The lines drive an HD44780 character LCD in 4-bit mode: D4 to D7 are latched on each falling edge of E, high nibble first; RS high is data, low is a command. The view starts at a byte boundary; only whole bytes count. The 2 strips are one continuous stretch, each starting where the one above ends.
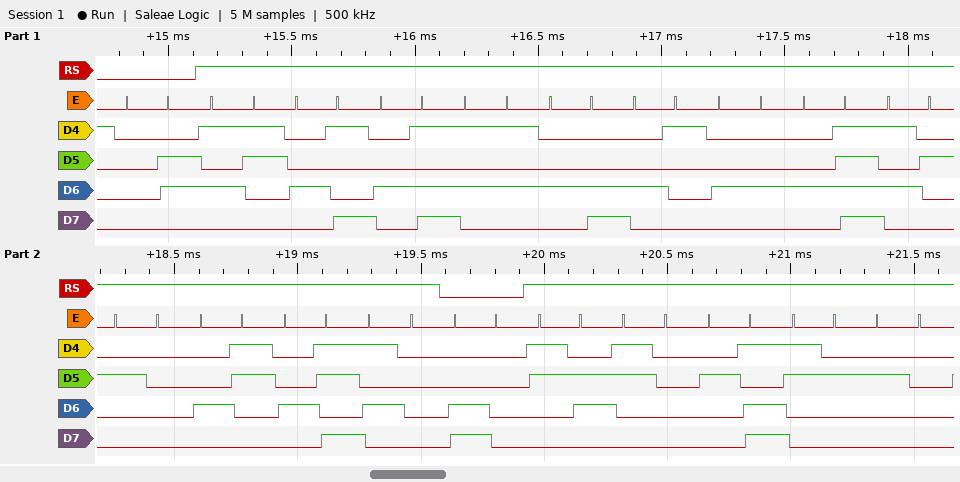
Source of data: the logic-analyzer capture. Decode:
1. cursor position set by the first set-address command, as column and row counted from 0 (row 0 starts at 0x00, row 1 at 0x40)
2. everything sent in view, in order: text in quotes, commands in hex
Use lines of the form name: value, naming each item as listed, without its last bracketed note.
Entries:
cursor position set by the first set-address command, as column and row counted from 0: column 0, row 1
everything sent in view, in order: text in quotes, commands in hex: 0x06 "SIMULADOR CKP" 0xC0 "60-2 "
